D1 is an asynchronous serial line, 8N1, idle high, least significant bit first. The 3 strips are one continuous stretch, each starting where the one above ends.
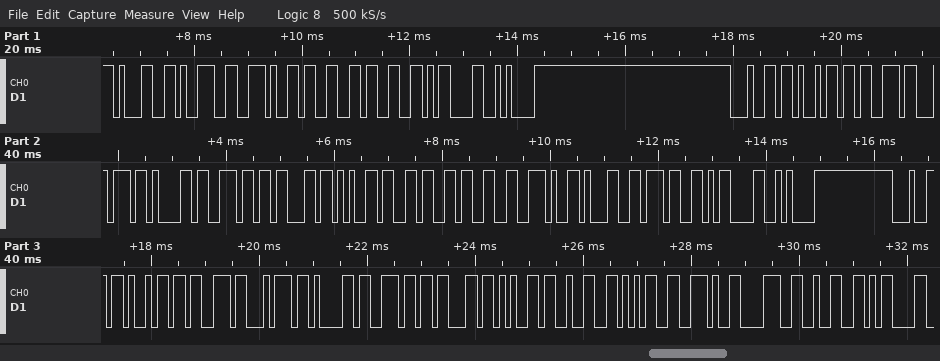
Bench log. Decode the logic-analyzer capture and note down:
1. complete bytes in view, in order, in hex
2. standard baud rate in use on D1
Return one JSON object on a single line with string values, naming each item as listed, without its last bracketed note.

{"complete bytes in view, in order, in hex": "31 39 2E 33 33 0D 0A 64 69 73 74 61 6E 63 65 36 33 2E 31 37 0D 0A 64 69 73 74 61 6E 63 65 32 35 2E 38 32 0D", "standard baud rate in use on D1": "9600 baud"}
